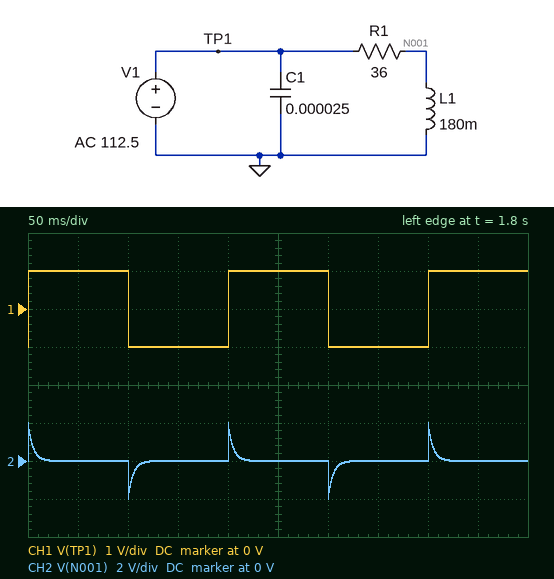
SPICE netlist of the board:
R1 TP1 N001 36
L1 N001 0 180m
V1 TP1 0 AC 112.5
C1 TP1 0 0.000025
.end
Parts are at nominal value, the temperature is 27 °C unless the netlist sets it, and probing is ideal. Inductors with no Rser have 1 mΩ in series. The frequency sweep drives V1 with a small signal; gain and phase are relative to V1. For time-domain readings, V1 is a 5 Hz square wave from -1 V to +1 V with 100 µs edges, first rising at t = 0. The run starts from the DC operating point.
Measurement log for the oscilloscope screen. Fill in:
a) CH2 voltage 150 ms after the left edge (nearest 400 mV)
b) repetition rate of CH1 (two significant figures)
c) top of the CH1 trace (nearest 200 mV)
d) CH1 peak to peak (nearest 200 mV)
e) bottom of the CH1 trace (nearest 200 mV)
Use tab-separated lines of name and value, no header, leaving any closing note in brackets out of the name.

CH2 voltage 150 ms after the left edge	0 V
repetition rate of CH1	5.0 Hz
top of the CH1 trace	1.0 V
CH1 peak to peak	2.0 V
bottom of the CH1 trace	-1.0 V
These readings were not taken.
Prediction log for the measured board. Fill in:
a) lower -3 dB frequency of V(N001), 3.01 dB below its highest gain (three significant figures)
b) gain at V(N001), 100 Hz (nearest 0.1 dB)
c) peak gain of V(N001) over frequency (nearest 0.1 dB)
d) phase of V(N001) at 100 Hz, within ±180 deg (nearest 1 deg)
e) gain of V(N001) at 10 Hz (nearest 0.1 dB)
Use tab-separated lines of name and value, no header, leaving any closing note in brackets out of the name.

lower -3 dB frequency of V(N001), 3.01 dB below its highest gain	31.8 Hz
gain at V(N001), 100 Hz	-0.4 dB
peak gain of V(N001) over frequency	0 dB
phase of V(N001) at 100 Hz, within ±180 deg	18 deg
gain of V(N001) at 10 Hz	-10.5 dB
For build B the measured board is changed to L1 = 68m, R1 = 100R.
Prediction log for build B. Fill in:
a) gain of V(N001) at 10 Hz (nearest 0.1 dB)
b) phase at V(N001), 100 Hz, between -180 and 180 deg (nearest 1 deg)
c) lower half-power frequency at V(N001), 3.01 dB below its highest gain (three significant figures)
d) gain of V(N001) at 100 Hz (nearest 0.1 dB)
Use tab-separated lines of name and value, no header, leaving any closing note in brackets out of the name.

gain of V(N001) at 10 Hz	-27.4 dB
phase at V(N001), 100 Hz, between -180 and 180 deg	67 deg
lower half-power frequency at V(N001), 3.01 dB below its highest gain	234 Hz
gain of V(N001) at 100 Hz	-8.1 dB
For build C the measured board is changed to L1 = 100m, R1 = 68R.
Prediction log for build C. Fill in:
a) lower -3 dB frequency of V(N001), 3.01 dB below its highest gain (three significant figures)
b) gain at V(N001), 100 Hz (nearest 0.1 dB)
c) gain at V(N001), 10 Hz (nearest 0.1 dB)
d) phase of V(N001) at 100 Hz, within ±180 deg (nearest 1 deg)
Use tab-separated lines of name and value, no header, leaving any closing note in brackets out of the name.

lower -3 dB frequency of V(N001), 3.01 dB below its highest gain	108 Hz
gain at V(N001), 100 Hz	-3.4 dB
gain at V(N001), 10 Hz	-20.7 dB
phase of V(N001) at 100 Hz, within ±180 deg	47 deg
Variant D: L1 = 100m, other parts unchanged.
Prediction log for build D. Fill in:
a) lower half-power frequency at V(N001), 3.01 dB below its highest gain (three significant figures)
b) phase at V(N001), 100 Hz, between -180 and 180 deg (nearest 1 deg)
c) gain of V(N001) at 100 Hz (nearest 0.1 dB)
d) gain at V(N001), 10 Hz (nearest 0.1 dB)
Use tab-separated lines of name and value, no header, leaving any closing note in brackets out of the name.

lower half-power frequency at V(N001), 3.01 dB below its highest gain	57.3 Hz
phase at V(N001), 100 Hz, between -180 and 180 deg	30 deg
gain of V(N001) at 100 Hz	-1.2 dB
gain at V(N001), 10 Hz	-15.3 dB
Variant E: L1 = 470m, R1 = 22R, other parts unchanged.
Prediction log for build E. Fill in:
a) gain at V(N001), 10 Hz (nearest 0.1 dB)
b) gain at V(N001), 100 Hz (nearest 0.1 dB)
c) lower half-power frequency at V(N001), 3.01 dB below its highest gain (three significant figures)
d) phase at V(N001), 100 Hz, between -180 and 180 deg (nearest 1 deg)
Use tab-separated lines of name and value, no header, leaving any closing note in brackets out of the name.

gain at V(N001), 10 Hz	-1.9 dB
gain at V(N001), 100 Hz	0 dB
lower half-power frequency at V(N001), 3.01 dB below its highest gain	7.45 Hz
phase at V(N001), 100 Hz, between -180 and 180 deg	4 deg
